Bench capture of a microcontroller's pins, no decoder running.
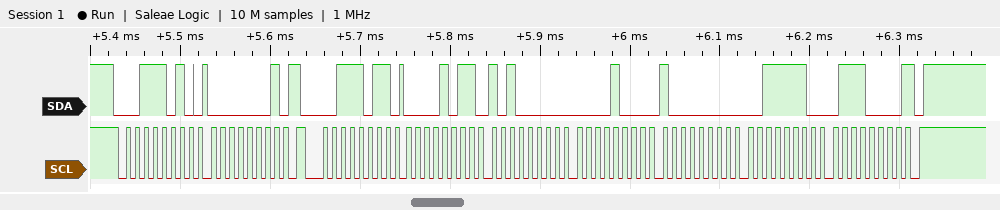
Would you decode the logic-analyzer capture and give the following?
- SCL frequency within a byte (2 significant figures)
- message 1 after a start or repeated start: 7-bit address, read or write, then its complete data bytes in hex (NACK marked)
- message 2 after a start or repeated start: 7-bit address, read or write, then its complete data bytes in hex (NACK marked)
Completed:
100 kHz
0x1D write: 01
0x1D read: 0B A0 08 80 3E 70 NACK
